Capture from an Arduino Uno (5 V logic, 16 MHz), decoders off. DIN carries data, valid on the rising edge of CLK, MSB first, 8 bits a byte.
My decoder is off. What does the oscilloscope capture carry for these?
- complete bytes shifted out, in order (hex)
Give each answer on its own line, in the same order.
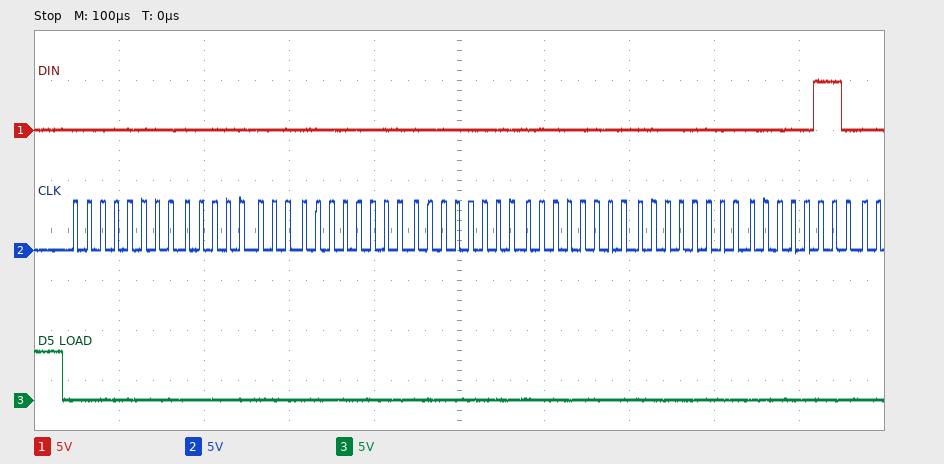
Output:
00 00 00 00 00 00 06
